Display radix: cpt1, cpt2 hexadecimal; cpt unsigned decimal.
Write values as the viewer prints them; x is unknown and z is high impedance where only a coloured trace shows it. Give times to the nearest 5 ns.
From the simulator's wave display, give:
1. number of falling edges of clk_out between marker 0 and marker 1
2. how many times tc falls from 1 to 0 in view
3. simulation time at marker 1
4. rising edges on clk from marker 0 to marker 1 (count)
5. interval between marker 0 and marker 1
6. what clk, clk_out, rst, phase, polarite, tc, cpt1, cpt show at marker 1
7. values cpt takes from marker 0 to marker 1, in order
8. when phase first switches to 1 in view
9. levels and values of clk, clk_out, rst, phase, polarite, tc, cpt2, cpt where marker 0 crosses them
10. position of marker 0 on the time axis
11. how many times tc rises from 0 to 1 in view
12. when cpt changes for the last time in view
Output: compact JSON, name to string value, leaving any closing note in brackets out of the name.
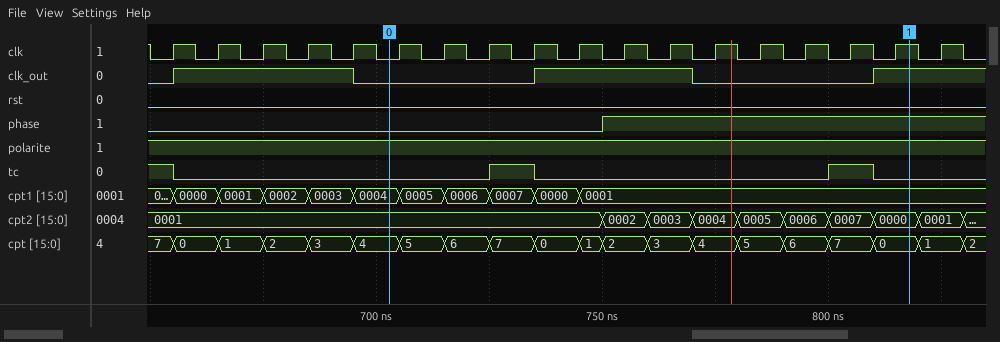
{"number of falling edges of clk_out between marker 0 and marker 1": "1", "how many times tc falls from 1 to 0 in view": "3", "simulation time at marker 1": "820 ns", "rising edges on clk from marker 0 to marker 1": "12", "interval between marker 0 and marker 1": "115 ns", "what clk, clk_out, rst, phase, polarite, tc, cpt1, cpt show at marker 1": "clk=1, clk_out=1, rst=0, phase=1, polarite=1, tc=0, cpt1=0001, cpt=0", "values cpt takes from marker 0 to marker 1, in order": "4, 5, 6, 7, 0, 1, 2, 3, 4, 5, 6, 7, 0", "when phase first switches to 1 in view": "750 ns", "levels and values of clk, clk_out, rst, phase, polarite, tc, cpt2, cpt where marker 0 crosses them": "clk=0, clk_out=0, rst=0, phase=0, polarite=1, tc=0, cpt2=0001, cpt=4", "position of marker 0 on the time axis": "705 ns", "how many times tc rises from 0 to 1 in view": "2", "when cpt changes for the last time in view": "830 ns"}
